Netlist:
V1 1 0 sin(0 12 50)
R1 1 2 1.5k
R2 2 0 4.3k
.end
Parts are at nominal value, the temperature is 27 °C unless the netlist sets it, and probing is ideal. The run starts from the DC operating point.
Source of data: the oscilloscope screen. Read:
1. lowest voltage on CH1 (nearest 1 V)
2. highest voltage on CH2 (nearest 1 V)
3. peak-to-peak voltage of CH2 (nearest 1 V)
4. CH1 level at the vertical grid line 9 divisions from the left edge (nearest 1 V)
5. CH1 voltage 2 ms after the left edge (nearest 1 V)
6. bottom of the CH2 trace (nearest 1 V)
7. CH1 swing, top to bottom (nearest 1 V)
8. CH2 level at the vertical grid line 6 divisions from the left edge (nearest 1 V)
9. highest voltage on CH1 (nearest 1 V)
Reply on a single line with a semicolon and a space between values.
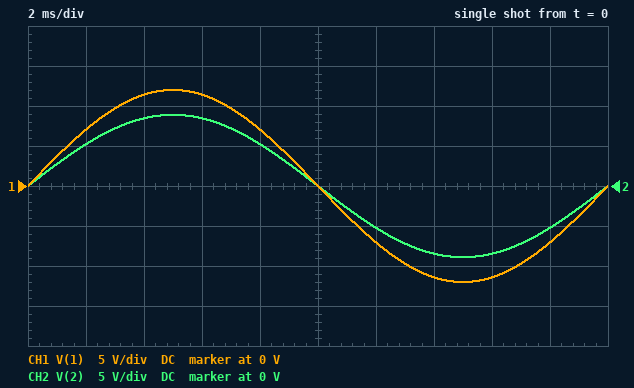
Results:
-12 V; 9 V; 18 V; -7 V; 7 V; -9 V; 24 V; -5 V; 12 V
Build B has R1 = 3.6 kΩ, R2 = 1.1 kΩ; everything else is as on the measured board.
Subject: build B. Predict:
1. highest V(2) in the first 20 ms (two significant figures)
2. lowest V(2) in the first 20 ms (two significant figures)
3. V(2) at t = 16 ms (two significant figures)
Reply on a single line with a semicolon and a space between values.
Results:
2.8 V; -2.8 V; -2.7 V
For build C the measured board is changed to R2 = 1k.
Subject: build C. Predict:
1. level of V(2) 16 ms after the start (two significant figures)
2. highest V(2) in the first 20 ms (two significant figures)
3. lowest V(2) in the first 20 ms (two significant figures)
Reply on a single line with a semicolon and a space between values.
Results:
-4.6 V; 4.8 V; -4.8 V
